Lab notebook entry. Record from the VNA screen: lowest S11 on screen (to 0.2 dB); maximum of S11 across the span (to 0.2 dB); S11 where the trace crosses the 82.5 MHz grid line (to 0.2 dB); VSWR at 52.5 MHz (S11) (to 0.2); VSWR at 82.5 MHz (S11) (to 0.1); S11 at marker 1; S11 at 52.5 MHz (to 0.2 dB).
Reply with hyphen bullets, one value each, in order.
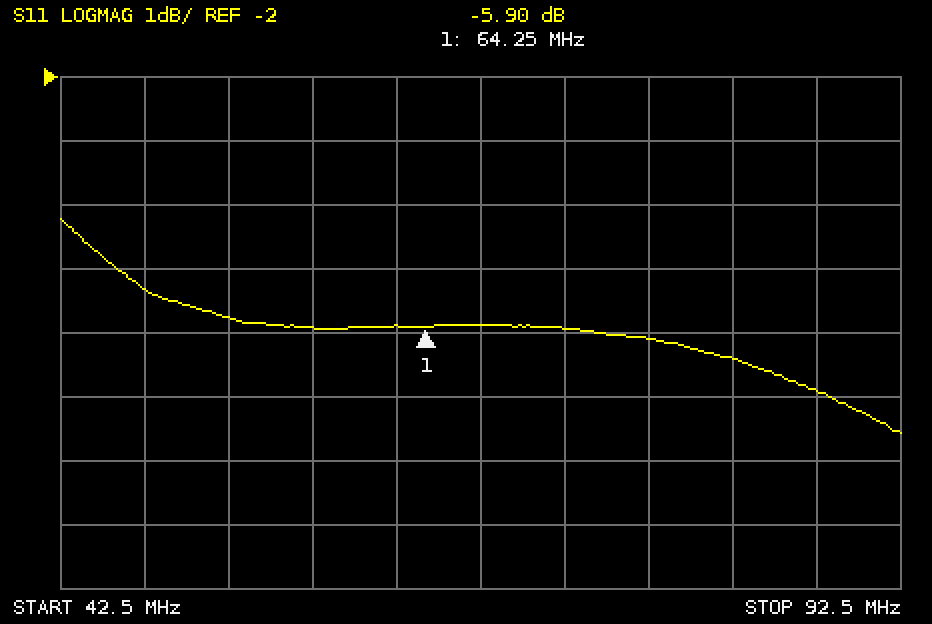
- -7.6 dB
- -4.2 dB
- -6.4 dB
- 3.2
- 2.8
- -5.90 dB
- -5.8 dB
